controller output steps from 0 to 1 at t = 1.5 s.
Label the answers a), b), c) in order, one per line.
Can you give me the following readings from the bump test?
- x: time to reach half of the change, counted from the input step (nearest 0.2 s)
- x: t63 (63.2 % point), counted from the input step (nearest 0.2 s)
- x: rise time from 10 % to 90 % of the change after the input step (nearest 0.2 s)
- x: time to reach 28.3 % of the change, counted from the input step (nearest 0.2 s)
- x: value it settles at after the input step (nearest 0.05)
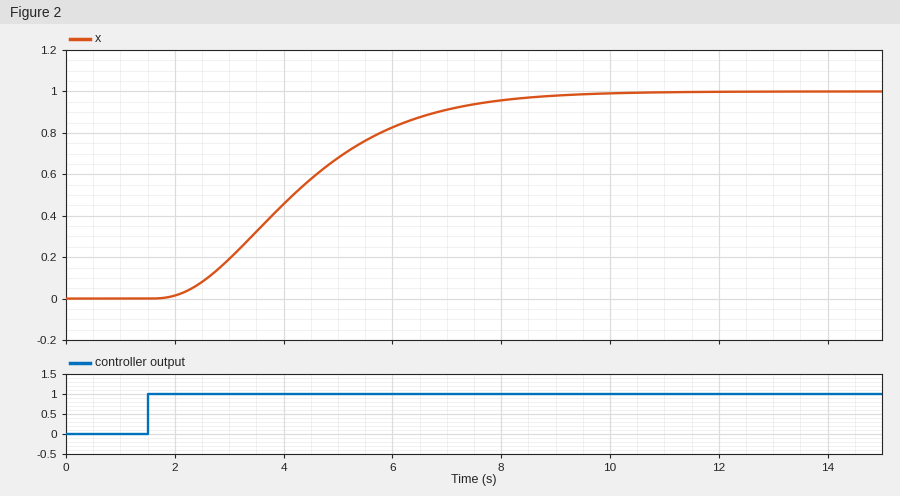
a) 2.6 s
b) 3.2 s
c) 4.2 s
d) 1.8 s
e) 1.00
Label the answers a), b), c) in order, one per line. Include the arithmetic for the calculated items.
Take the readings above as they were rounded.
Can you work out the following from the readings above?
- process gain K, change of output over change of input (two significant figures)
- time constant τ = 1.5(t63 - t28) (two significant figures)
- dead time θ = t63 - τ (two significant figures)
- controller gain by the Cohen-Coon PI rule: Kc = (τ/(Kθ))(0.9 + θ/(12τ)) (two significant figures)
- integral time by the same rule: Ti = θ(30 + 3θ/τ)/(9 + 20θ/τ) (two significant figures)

a) (1 - 0) / 1 = 1.0
b) 1.5 × (3.2 - 1.8) = 2.1 s
c) 3.2 - 2.1 = 1.1 s
d) 2.1 / (1 × 1.1) × (0.9 + 1.1 / (12 × 2.1)) = 1.8
e) 1.1 × (30 + 3 × 1.1 / 2.1) / (9 + 20 × 1.1 / 2.1) = 1.8 s
